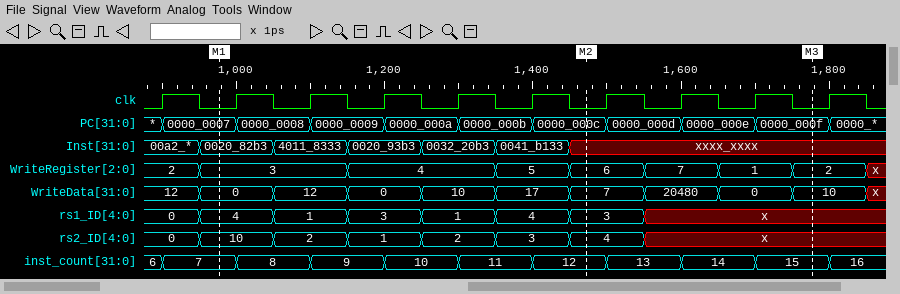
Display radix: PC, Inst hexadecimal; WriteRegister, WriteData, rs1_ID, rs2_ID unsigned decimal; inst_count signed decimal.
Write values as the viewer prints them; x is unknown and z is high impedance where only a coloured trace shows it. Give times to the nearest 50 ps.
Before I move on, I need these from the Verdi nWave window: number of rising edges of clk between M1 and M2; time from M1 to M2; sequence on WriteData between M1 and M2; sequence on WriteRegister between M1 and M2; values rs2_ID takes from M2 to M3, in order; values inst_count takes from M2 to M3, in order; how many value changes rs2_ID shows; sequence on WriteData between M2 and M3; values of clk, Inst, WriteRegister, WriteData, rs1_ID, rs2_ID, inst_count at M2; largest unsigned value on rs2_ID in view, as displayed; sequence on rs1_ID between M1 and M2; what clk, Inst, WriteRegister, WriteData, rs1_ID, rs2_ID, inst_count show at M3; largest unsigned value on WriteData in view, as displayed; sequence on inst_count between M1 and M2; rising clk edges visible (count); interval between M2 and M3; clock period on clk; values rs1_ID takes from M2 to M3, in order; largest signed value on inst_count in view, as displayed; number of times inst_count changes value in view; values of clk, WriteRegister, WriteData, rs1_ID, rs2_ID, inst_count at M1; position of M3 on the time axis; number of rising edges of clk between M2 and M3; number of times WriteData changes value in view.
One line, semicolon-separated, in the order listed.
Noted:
5; 500 ps; 0, 12, 0, 10, 17, 7; 3, 4, 5, 6; 4, x; 12, 13, 14, 15; 7; 7, 20480, 0, 10; clk=0, Inst=xxxx_xxxx, WriteRegister=6, WriteData=7, rs1_ID=3, rs2_ID=4, inst_count=12; 10; 4, 1, 3, 1, 4, 3; clk=0, Inst=xxxx_xxxx, WriteRegister=2, WriteData=10, rs1_ID=x, rs2_ID=x, inst_count=15; 20480; 7, 8, 9, 10, 11, 12; 10; 300 ps; 100 ps; 3, x; 16; 10; clk=0, WriteRegister=3, WriteData=0, rs1_ID=4, rs2_ID=10, inst_count=7; 1800 ps; 3; 10
